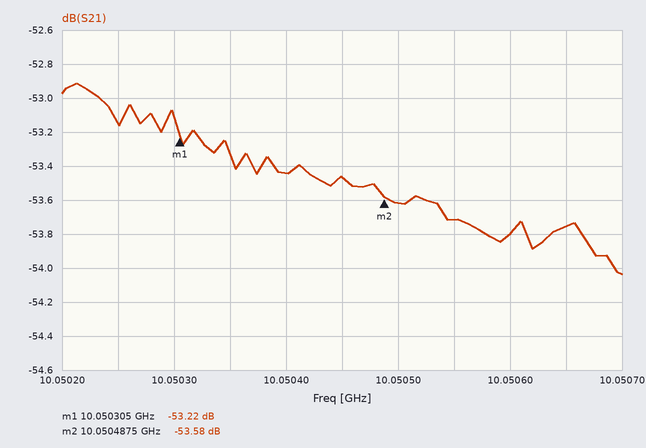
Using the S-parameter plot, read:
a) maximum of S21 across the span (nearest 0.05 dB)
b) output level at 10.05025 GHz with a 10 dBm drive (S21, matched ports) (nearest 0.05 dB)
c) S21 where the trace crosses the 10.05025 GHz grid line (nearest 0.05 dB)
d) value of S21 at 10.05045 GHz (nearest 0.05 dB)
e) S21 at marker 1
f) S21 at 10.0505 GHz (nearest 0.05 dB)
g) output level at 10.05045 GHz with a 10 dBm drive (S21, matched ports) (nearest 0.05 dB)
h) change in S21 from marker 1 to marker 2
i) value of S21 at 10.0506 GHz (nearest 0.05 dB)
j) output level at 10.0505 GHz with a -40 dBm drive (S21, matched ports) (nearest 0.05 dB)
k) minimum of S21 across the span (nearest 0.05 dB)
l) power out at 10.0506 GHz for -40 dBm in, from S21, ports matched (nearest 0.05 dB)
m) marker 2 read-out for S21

-52.90 dB
-43.15 dBm
-53.15 dB
-53.45 dB
-53.22 dB
-53.60 dB
-43.45 dBm
-0.36 dB
-53.80 dB
-93.60 dBm
-54.05 dB
-93.80 dBm
-53.58 dB
